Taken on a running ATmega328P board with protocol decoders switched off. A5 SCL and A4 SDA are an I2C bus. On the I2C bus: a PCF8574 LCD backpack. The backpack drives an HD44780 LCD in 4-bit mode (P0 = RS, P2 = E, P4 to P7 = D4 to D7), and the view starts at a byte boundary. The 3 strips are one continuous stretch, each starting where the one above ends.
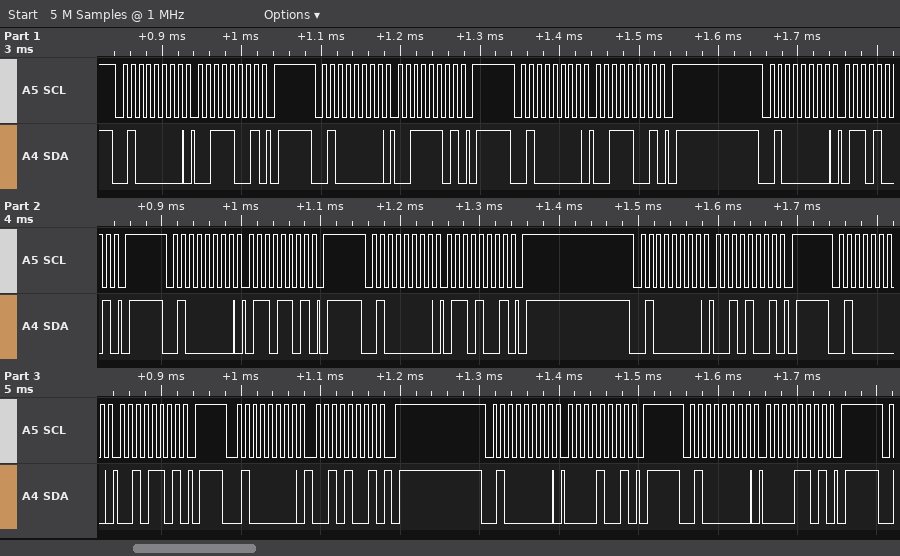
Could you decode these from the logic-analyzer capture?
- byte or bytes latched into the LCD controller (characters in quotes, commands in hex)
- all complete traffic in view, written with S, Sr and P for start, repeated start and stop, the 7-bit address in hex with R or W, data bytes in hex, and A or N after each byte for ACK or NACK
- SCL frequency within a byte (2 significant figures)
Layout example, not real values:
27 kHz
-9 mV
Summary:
'6'
S 20W A 39 A P S 20W A 3D A P S 20W A 39 A P S 20W A 69 A P S 20W A 6D A P S 20W A 69 A P S 20W A 29 A P S 20W A 2D A P S 20W A 29 A P S 20W A 09 A P S 20W A 0D A P
100 kHz
